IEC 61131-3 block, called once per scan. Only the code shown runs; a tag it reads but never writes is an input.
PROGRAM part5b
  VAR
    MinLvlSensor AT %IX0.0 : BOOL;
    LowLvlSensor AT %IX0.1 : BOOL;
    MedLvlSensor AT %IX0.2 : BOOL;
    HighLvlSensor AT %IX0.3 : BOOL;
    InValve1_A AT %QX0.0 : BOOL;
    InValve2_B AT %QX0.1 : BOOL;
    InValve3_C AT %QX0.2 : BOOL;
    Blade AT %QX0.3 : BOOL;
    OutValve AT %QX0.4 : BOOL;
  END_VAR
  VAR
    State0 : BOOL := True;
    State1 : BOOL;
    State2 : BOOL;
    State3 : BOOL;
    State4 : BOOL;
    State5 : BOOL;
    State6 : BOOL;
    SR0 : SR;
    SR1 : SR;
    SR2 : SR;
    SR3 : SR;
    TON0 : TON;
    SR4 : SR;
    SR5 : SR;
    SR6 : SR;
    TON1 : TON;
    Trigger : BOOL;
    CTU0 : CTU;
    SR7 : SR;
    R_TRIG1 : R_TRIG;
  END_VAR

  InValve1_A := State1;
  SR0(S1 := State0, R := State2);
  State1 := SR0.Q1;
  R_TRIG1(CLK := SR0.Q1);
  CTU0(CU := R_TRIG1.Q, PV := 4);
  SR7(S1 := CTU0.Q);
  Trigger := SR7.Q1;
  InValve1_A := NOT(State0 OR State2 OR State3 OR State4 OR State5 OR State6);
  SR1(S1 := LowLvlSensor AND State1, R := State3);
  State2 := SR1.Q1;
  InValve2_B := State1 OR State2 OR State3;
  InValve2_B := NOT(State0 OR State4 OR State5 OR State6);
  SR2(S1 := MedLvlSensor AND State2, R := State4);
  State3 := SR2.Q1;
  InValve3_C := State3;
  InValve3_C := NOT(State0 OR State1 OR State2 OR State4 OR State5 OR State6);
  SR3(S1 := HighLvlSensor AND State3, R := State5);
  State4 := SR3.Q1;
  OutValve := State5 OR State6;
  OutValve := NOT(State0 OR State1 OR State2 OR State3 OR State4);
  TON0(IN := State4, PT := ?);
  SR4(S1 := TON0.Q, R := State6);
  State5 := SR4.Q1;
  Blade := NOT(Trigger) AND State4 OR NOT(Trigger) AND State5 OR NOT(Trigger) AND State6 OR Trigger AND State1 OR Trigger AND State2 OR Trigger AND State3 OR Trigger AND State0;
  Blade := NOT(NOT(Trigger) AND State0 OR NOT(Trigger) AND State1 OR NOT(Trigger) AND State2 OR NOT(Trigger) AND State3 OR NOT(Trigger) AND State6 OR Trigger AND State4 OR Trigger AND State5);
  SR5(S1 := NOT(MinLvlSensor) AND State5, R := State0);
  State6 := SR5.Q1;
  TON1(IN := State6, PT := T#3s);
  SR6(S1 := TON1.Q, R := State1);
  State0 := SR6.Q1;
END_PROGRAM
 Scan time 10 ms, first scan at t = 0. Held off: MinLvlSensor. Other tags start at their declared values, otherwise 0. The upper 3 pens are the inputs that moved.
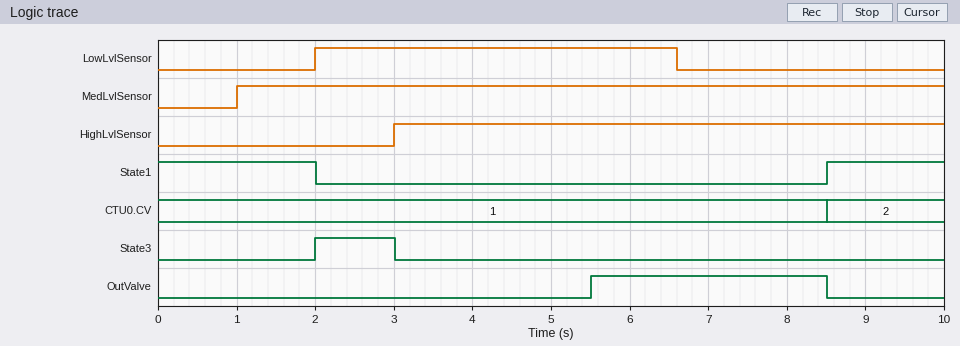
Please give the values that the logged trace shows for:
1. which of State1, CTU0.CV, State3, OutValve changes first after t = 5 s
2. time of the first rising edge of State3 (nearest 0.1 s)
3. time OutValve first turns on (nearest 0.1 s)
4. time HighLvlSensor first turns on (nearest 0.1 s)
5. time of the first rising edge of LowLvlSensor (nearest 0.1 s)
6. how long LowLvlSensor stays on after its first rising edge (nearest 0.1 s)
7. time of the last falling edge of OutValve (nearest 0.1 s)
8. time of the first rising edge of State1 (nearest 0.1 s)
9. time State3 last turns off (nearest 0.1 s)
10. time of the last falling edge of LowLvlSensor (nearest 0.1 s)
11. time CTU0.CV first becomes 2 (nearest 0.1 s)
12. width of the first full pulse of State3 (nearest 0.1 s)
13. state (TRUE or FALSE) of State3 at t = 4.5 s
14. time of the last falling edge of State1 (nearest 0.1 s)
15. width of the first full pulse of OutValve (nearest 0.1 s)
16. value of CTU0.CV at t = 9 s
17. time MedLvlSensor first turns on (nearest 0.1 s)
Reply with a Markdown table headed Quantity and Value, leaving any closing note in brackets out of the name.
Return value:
| Quantity | Value |
|---|---|
| which of State1, CTU0.CV, State3, OutValve changes first after t = 5 s | OutValve |
| time of the first rising edge of State3 | 2.0 s |
| time OutValve first turns on | 5.5 s |
| time HighLvlSensor first turns on | 3.0 s |
| time of the first rising edge of LowLvlSensor | 2.0 s |
| how long LowLvlSensor stays on after its first rising edge | 4.6 s |
| time of the last falling edge of OutValve | 8.5 s |
| time of the first rising edge of State1 | 8.5 s |
| time State3 last turns off | 3.0 s |
| time of the last falling edge of LowLvlSensor | 6.6 s |
| time CTU0.CV first becomes 2 | 8.5 s |
| width of the first full pulse of State3 | 1.0 s |
| state (TRUE or FALSE) of State3 at t = 4.5 s | FALSE |
| time of the last falling edge of State1 | 2.0 s |
| width of the first full pulse of OutValve | 3.0 s |
| value of CTU0.CV at t = 9 s | 2 |
| time MedLvlSensor first turns on | 1.0 s |
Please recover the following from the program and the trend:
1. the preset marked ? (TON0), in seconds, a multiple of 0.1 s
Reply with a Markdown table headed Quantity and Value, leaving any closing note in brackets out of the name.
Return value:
| Quantity | Value |
|---|---|
| the preset marked ? (TON0), in seconds, a multiple of 0.1 s | 2.5 s |
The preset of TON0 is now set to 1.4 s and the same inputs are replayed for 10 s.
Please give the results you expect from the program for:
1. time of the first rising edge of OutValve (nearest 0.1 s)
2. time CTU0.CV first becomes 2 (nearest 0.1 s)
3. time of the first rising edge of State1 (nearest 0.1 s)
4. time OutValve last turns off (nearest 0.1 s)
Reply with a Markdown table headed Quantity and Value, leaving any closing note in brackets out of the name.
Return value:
| Quantity | Value |
|---|---|
| time of the first rising edge of OutValve | 4.4 s |
| time CTU0.CV first becomes 2 | 7.4 s |
| time of the first rising edge of State1 | 7.4 s |
| time OutValve last turns off | 7.4 s |
